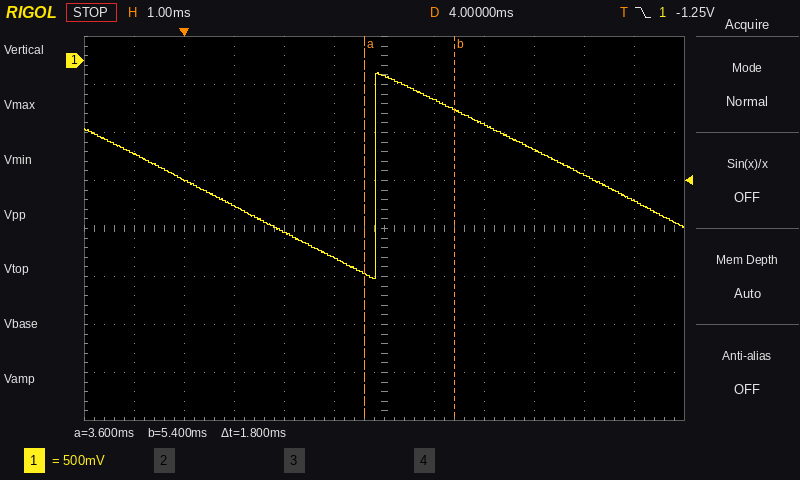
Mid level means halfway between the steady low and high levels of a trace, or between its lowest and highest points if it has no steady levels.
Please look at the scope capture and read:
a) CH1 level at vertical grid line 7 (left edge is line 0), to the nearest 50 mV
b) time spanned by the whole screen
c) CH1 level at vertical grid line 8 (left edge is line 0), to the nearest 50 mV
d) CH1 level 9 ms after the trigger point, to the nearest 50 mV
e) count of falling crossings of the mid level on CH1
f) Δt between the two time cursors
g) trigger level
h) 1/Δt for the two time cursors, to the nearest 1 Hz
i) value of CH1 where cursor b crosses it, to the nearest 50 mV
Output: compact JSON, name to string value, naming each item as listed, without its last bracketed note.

{"CH1 level at vertical grid line 7 (left edge is line 0), to the nearest 50 mV": "-400 mV", "time spanned by the whole screen": "12 ms", "CH1 level at vertical grid line 8 (left edge is line 0), to the nearest 50 mV": "-650 mV", "CH1 level 9 ms after the trigger point, to the nearest 50 mV": "-1.45 V", "count of falling crossings of the mid level on CH1": "2", "Δt between the two time cursors": "1.8 ms", "trigger level": "-1.25 V", "1/Δt for the two time cursors, to the nearest 1 Hz": "556 Hz", "value of CH1 where cursor b crosses it, to the nearest 50 mV": "-500 mV"}
